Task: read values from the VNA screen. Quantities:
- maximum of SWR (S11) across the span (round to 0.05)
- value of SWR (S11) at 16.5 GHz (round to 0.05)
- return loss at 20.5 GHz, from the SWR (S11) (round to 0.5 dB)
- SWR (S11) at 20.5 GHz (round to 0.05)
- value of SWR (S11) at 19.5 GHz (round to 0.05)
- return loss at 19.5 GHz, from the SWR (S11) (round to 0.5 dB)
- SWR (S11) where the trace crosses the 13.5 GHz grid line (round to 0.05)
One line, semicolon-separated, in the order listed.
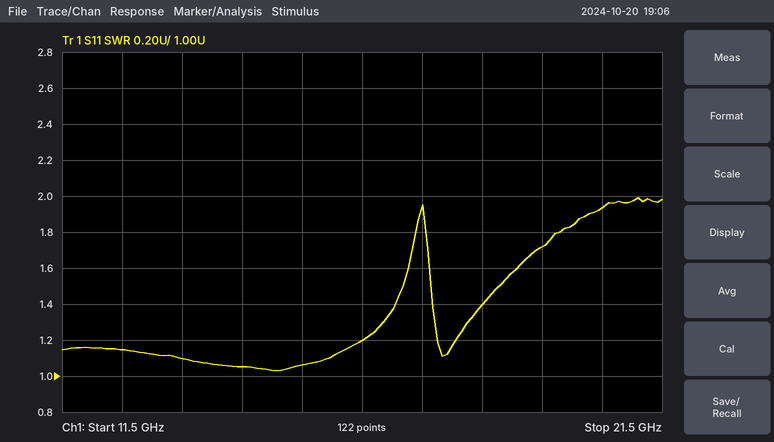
2.00; 1.20; 10.0 dB; 1.95; 1.70; 11.5 dB; 1.10
